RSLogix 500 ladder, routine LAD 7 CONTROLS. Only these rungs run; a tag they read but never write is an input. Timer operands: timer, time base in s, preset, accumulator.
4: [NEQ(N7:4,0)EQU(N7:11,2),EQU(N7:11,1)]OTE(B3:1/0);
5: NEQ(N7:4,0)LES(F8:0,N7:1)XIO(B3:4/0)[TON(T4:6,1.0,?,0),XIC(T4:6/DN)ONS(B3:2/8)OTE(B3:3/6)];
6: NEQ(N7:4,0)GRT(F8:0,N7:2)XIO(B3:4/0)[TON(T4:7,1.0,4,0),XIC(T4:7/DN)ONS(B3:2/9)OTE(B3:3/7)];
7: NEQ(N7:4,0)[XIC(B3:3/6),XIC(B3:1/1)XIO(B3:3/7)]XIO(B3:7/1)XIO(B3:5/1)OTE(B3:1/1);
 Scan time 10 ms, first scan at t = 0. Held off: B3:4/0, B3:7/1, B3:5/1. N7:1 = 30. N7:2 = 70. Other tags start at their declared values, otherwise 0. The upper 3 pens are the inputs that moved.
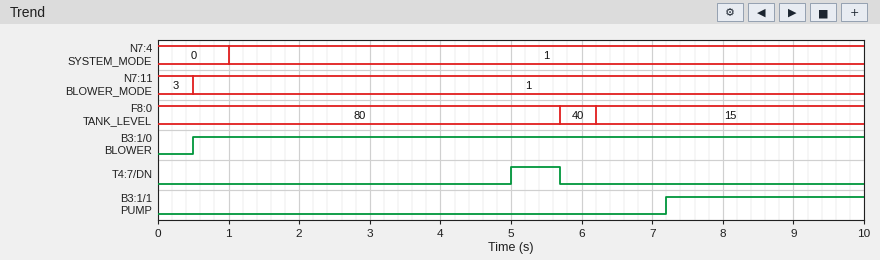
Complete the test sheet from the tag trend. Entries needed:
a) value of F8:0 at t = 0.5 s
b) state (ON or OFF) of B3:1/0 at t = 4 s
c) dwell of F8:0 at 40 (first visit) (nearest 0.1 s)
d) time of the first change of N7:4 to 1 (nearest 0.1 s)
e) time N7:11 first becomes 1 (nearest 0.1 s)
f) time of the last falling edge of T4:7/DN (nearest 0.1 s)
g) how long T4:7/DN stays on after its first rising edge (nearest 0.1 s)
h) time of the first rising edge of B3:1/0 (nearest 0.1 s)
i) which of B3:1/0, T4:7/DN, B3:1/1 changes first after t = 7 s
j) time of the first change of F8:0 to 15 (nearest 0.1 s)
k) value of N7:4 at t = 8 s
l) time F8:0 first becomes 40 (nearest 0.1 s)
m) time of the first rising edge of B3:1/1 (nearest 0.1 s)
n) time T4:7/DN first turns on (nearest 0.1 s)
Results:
80
ON
0.5 s
1.0 s
0.5 s
5.7 s
0.7 s
0.5 s
B3:1/1
6.2 s
1
5.7 s
7.2 s
5.0 s
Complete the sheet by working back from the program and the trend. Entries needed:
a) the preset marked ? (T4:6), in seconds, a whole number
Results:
1 s
